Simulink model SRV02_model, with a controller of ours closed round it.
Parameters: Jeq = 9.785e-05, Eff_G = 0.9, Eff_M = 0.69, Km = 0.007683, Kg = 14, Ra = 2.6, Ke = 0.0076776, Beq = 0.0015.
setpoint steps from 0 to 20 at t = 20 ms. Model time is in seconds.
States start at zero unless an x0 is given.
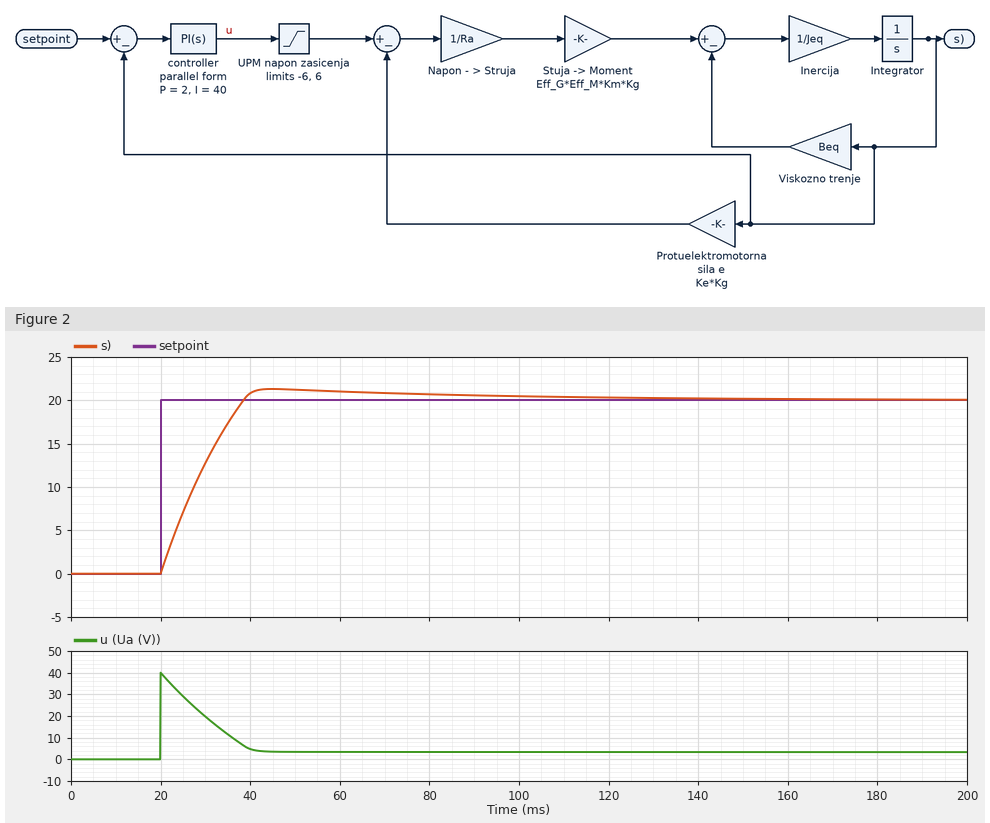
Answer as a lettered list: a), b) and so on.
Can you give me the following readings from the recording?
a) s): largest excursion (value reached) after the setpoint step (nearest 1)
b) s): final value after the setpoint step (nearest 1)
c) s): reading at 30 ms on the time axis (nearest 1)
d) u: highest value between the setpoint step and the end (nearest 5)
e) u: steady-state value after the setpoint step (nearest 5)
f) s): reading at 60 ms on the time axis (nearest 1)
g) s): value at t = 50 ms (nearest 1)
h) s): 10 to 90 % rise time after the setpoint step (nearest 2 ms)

a) 21
b) 20
c) 13
d) 40
e) 5
f) 21
g) 21
h) 14 ms
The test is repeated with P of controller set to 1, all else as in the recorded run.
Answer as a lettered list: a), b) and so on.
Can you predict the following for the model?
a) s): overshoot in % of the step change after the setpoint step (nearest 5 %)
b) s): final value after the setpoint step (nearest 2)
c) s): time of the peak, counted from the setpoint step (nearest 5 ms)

a) 10 %
b) 20
c) 25 ms
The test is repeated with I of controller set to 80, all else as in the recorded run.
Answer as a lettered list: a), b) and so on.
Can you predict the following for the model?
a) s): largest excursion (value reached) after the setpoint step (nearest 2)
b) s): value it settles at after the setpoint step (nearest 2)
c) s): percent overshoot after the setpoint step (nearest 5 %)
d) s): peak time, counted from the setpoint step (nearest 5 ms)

a) 24
b) 20
c) 20 %
d) 25 ms
